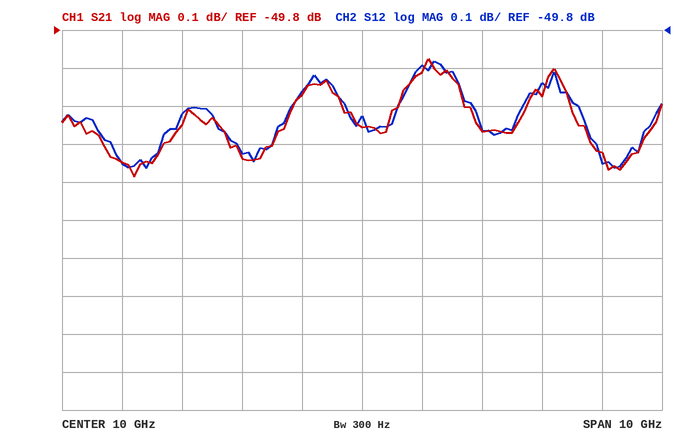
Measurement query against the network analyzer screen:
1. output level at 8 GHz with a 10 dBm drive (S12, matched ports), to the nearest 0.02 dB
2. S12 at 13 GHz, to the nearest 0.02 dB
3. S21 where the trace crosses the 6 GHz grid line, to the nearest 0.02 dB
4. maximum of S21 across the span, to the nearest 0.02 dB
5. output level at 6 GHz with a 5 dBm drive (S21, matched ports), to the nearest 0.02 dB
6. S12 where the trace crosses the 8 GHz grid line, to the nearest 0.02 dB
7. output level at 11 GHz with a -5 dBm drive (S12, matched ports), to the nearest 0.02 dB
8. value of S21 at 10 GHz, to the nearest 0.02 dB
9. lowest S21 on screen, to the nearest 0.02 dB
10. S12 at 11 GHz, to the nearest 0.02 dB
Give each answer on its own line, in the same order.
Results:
-40.12 dBm
-49.94 dB
-50.14 dB
-49.88 dB
-45.14 dBm
-50.12 dB
-54.90 dBm
-50.06 dB
-50.18 dB
-49.90 dB
